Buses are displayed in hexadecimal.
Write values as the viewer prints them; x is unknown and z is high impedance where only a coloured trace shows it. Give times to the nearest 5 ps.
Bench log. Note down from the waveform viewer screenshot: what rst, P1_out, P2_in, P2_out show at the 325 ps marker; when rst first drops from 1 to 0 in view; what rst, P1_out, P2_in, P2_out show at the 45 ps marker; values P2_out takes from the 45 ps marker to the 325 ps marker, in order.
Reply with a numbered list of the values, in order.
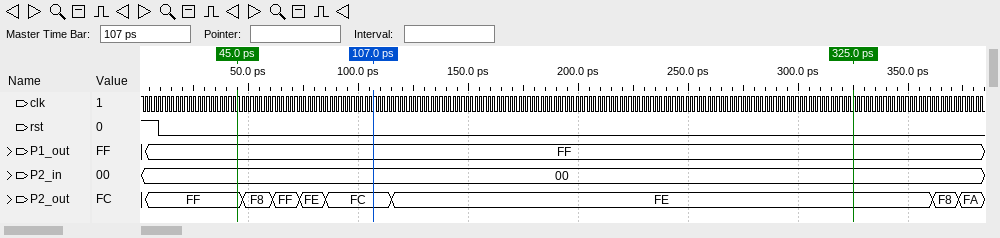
1. rst=0, P1_out=FF, P2_in=00, P2_out=FE
2. 10 ps
3. rst=0, P1_out=FF, P2_in=00, P2_out=FF
4. FF, F8, FF, FE, FC, FE
